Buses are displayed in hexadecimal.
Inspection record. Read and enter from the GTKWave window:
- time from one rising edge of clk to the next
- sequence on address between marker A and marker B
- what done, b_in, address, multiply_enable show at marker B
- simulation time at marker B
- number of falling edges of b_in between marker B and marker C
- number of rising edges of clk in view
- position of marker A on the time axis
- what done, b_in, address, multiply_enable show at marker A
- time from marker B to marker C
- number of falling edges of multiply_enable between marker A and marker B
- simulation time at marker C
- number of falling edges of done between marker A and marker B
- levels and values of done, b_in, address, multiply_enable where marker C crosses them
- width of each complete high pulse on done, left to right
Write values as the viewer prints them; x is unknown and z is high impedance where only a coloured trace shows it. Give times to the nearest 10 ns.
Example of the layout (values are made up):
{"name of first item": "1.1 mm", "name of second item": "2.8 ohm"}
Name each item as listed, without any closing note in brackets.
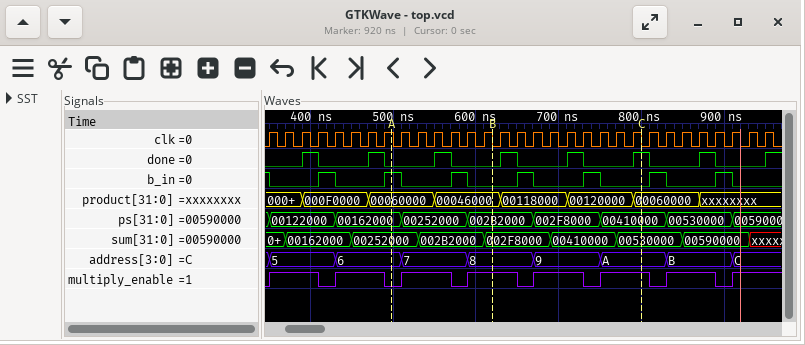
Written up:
{"time from one rising edge of clk to the next": "20 ns", "sequence on address between marker A and marker B": "6, 7, 8", "what done, b_in, address, multiply_enable show at marker B": "done=0, b_in=0, address=8, multiply_enable=1", "simulation time at marker B": "620 ns", "number of falling edges of b_in between marker B and marker C": "2", "number of rising edges of clk in view": "31", "position of marker A on the time axis": "500 ns", "what done, b_in, address, multiply_enable show at marker A": "done=0, b_in=1, address=6, multiply_enable=0", "time from marker B to marker C": "180 ns", "number of falling edges of multiply_enable between marker A and marker B": "1", "simulation time at marker C": "800 ns", "number of falling edges of done between marker A and marker B": "1", "levels and values of done, b_in, address, multiply_enable where marker C crosses them": "done=1, b_in=0, address=A, multiply_enable=1", "width of each complete high pulse on done, left to right": "20 ns, 20 ns, 20 ns, 20 ns, 20 ns, 20 ns, 20 ns"}
